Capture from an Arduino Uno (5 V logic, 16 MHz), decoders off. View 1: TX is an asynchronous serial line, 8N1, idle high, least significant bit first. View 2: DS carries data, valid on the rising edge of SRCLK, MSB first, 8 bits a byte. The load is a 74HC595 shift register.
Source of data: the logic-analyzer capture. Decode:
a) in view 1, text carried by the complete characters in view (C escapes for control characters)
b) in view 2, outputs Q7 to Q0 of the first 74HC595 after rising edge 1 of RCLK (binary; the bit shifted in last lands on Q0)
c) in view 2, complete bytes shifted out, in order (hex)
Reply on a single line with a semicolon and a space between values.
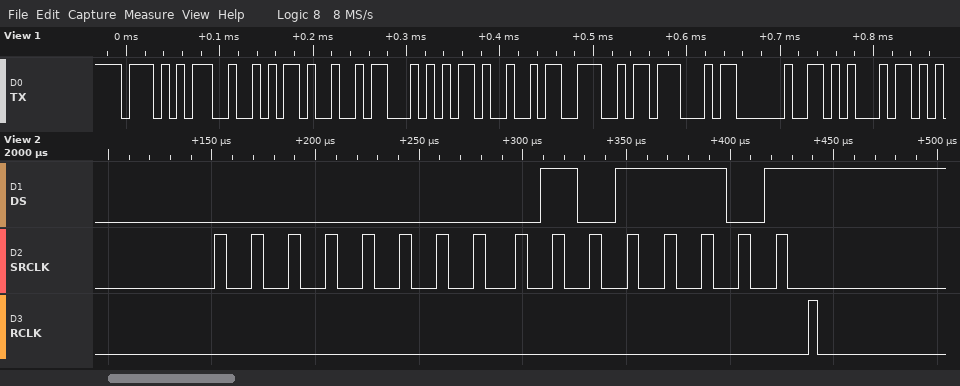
"WRITING E"; 01011101; 00 5D
